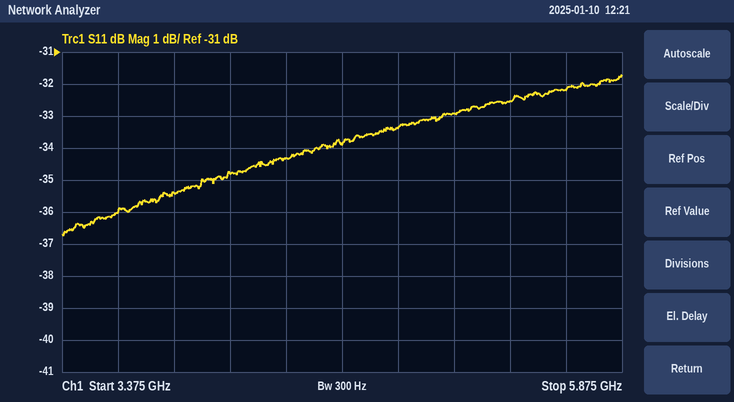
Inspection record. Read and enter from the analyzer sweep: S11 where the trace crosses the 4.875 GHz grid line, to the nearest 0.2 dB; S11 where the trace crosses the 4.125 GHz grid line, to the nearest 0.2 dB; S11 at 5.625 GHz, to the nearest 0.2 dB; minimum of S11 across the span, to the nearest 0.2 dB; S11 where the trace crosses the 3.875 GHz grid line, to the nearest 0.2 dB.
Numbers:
-33.4 dB
-34.8 dB
-32.2 dB
-36.8 dB
-35.4 dB
